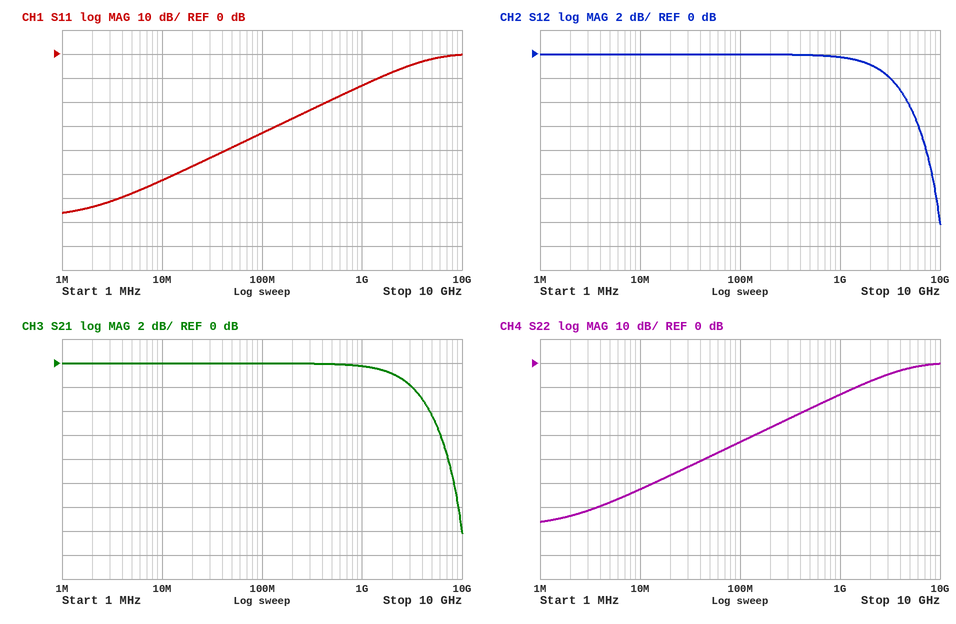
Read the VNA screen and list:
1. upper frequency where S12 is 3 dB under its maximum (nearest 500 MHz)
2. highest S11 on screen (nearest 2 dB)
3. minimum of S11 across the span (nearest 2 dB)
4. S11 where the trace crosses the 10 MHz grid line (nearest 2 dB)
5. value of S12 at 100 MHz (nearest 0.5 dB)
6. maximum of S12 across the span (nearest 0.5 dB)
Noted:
4.0 GHz
0 dB
-66 dB
-52 dB
0.0 dB
0.0 dB
